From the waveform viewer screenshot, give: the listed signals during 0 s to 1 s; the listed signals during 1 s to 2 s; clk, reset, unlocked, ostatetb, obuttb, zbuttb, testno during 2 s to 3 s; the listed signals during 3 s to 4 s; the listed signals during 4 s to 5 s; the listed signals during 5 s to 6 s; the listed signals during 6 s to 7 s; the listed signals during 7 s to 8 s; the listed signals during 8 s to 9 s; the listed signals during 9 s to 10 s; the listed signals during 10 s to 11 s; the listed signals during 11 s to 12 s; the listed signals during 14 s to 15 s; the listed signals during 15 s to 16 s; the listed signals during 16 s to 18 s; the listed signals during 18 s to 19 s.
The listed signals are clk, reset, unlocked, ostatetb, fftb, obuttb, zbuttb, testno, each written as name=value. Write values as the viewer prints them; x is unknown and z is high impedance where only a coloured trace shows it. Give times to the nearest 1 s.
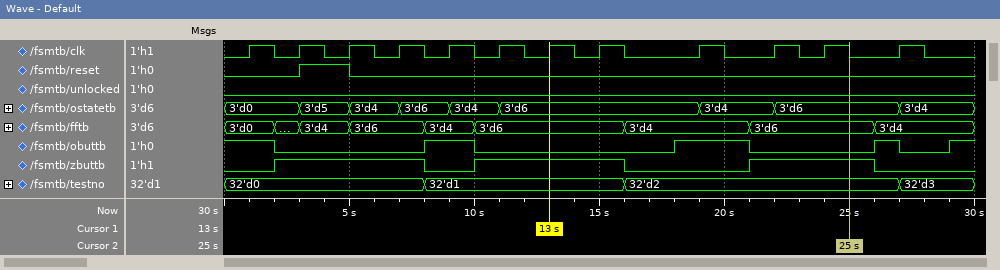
clk=0, reset=0, unlocked=0, ostatetb=3'd0, fftb=3'd0, obuttb=1, zbuttb=0, testno=32'd0
clk=1, reset=0, unlocked=0, ostatetb=3'd0, fftb=3'd0, obuttb=1, zbuttb=0, testno=32'd0
clk=0, reset=0, unlocked=0, ostatetb=3'd0, obuttb=0, zbuttb=1, testno=32'd0
clk=1, reset=1, unlocked=0, ostatetb=3'd5, fftb=3'd4, obuttb=0, zbuttb=1, testno=32'd0
clk=0, reset=1, unlocked=0, ostatetb=3'd5, fftb=3'd4, obuttb=0, zbuttb=1, testno=32'd0
clk=1, reset=0, unlocked=0, ostatetb=3'd4, fftb=3'd6, obuttb=0, zbuttb=1, testno=32'd0
clk=0, reset=0, unlocked=0, ostatetb=3'd4, fftb=3'd6, obuttb=0, zbuttb=1, testno=32'd0
clk=1, reset=0, unlocked=0, ostatetb=3'd6, fftb=3'd6, obuttb=0, zbuttb=1, testno=32'd0
clk=0, reset=0, unlocked=0, ostatetb=3'd6, fftb=3'd4, obuttb=1, zbuttb=0, testno=32'd1
clk=1, reset=0, unlocked=0, ostatetb=3'd4, fftb=3'd4, obuttb=1, zbuttb=0, testno=32'd1
clk=0, reset=0, unlocked=0, ostatetb=3'd4, fftb=3'd6, obuttb=0, zbuttb=1, testno=32'd1
clk=1, reset=0, unlocked=0, ostatetb=3'd6, fftb=3'd6, obuttb=0, zbuttb=1, testno=32'd1
clk=0, reset=0, unlocked=0, ostatetb=3'd6, fftb=3'd6, obuttb=0, zbuttb=1, testno=32'd1
clk=1, reset=0, unlocked=0, ostatetb=3'd6, fftb=3'd6, obuttb=0, zbuttb=1, testno=32'd1
clk=0, reset=0, unlocked=0, ostatetb=3'd6, fftb=3'd4, obuttb=0, zbuttb=0, testno=32'd2
clk=0, reset=0, unlocked=0, ostatetb=3'd6, fftb=3'd4, obuttb=1, zbuttb=0, testno=32'd2
